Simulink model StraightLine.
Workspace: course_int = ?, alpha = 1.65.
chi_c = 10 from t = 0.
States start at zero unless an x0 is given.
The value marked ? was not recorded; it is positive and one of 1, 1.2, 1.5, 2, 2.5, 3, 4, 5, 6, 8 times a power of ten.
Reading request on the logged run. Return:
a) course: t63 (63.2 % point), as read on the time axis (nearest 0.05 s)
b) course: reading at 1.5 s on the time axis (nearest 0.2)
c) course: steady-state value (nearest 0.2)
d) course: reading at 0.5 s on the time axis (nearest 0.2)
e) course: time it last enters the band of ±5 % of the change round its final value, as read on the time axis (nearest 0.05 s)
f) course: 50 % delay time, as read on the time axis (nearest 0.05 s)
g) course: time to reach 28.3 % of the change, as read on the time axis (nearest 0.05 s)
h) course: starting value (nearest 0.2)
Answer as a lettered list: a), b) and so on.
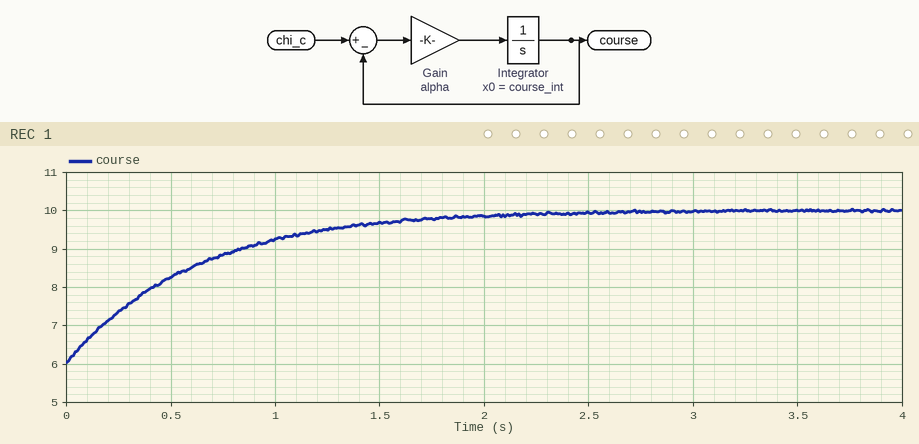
a) 0.60 s
b) 9.6
c) 10.0
d) 8.2
e) 1.80 s
f) 0.40 s
g) 0.20 s
h) 6.0
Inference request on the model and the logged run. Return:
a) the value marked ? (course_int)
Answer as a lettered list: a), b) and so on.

a) 6
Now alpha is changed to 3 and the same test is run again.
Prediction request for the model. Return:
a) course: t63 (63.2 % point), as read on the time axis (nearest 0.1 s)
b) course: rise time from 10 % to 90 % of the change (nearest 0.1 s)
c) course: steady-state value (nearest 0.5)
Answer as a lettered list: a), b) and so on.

a) 0.3 s
b) 0.7 s
c) 10.0
